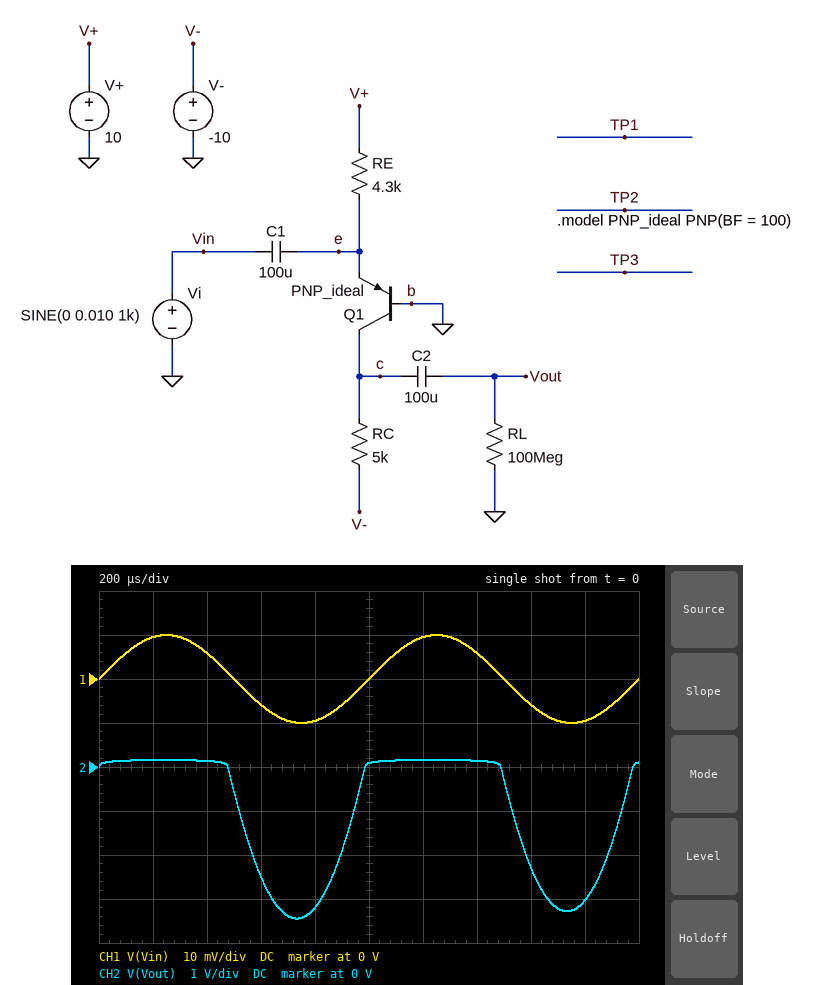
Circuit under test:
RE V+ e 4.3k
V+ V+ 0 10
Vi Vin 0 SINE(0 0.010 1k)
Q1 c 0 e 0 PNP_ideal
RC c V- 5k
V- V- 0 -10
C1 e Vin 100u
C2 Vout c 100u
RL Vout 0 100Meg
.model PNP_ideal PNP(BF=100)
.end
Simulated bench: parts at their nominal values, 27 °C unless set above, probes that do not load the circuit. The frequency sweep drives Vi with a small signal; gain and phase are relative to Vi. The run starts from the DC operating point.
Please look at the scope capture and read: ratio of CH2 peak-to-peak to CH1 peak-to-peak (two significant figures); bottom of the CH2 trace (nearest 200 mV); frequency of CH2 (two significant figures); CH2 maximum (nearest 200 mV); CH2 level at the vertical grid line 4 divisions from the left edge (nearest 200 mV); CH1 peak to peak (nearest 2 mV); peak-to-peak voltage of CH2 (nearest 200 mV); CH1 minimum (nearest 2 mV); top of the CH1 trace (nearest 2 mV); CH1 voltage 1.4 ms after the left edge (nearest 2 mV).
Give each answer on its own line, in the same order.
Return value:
180
-3.4 V
1.0 kHz
200 mV
-3.2 V
20 mV
3.6 V
-10 mV
10 mV
6 mV
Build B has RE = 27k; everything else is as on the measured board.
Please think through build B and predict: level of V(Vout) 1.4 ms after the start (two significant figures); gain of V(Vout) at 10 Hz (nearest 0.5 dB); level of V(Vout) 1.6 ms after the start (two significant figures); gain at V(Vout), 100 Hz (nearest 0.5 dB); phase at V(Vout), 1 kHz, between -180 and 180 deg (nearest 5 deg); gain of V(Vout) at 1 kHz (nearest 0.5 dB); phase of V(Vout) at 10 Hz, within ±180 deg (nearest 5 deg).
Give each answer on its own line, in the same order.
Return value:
390 mV
29.0 dB
-370 mV
36.0 dB
0 deg
36.5 dB
65 deg
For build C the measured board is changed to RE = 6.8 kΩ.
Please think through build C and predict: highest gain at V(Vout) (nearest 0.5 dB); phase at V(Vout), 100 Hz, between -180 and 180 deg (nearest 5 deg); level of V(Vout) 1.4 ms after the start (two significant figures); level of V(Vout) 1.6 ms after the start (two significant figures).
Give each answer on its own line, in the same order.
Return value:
48.5 dB
40 deg
1.2 V
-1.7 V
